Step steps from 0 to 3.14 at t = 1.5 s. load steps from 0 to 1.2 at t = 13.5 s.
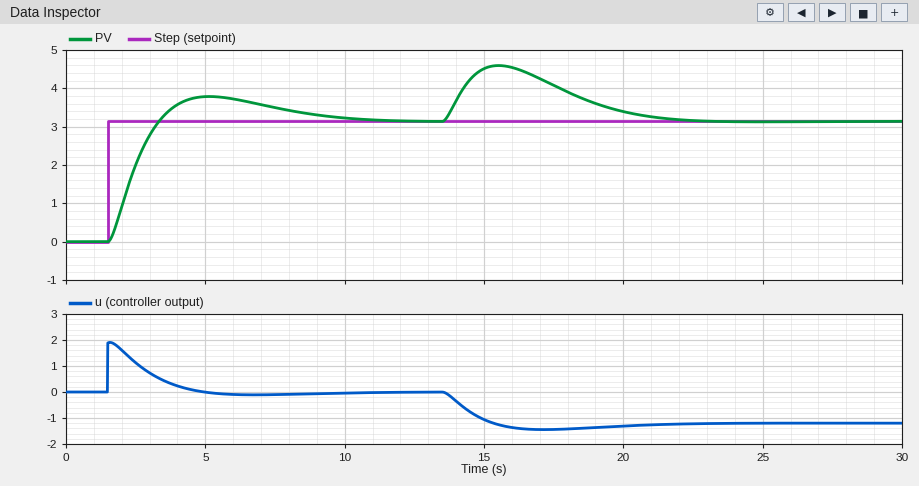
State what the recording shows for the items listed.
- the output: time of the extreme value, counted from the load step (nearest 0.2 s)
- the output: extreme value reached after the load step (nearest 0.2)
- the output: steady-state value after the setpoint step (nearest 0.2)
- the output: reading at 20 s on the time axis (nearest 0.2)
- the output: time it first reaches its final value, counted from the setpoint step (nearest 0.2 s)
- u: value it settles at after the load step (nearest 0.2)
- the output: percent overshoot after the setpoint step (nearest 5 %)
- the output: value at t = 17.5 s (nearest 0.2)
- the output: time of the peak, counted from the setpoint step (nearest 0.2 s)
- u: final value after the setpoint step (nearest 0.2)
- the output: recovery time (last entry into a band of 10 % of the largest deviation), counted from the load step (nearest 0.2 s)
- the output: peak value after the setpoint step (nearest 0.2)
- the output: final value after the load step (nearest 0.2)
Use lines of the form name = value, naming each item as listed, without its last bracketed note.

the output: time of the extreme value, counted from the load step = 2.0 s
the output: extreme value reached after the load step = 4.6
the output: steady-state value after the setpoint step = 3.2
the output: reading at 20 s on the time axis = 3.4
the output: time it first reaches its final value, counted from the setpoint step = 1.8 s
u: value it settles at after the load step = -1.2
the output: percent overshoot after the setpoint step = 20 %
the output: value at t = 17.5 s = 4.0
the output: time of the peak, counted from the setpoint step = 3.6 s
u: final value after the setpoint step = 0.0
the output: recovery time (last entry into a band of 10 % of the largest deviation), counted from the load step = 7.2 s
the output: peak value after the setpoint step = 3.8
the output: final value after the load step = 3.2
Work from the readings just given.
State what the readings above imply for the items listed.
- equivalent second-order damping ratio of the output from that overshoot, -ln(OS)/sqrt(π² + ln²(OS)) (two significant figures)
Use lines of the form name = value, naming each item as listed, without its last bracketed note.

equivalent second-order damping ratio of the output from that overshoot, -ln(OS)/sqrt(π² + ln²(OS)) = 0.46
